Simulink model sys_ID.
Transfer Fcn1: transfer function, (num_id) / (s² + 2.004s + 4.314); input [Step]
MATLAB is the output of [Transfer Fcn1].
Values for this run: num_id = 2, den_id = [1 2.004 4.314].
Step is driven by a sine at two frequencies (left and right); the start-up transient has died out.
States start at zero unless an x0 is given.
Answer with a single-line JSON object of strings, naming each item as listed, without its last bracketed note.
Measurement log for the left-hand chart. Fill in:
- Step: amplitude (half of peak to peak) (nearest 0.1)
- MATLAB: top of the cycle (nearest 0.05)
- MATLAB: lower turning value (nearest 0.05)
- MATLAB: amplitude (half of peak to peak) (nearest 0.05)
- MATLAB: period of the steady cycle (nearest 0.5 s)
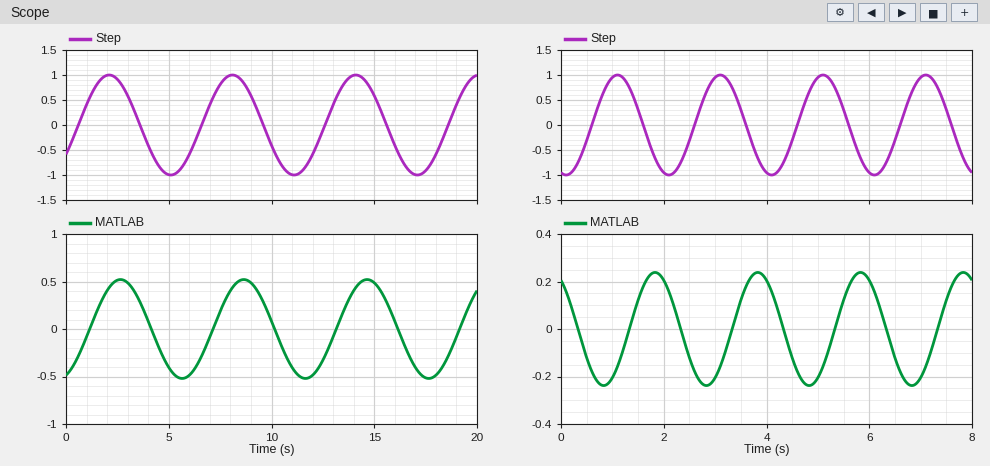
{"Step: amplitude (half of peak to peak)": "1.0", "MATLAB: top of the cycle": "0.50", "MATLAB: lower turning value": "-0.50", "MATLAB: amplitude (half of peak to peak)": "0.50", "MATLAB: period of the steady cycle": "6.0 s"}
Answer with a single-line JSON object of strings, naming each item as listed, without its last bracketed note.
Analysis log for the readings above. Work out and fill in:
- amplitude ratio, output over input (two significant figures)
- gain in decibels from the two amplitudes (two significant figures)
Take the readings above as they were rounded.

{"amplitude ratio, output over input": "0.50", "gain in decibels from the two amplitudes": "-6.0 dB"}
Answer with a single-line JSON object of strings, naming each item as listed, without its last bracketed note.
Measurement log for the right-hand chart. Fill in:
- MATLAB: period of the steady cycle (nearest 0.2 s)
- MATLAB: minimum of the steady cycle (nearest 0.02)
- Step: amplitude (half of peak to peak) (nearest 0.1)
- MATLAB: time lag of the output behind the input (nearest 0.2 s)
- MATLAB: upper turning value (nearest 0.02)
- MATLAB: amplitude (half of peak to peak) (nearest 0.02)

{"MATLAB: period of the steady cycle": "2.0 s", "MATLAB: minimum of the steady cycle": "-0.24", "Step: amplitude (half of peak to peak)": "1.0", "MATLAB: time lag of the output behind the input": "0.8 s", "MATLAB: upper turning value": "0.24", "MATLAB: amplitude (half of peak to peak)": "0.24"}
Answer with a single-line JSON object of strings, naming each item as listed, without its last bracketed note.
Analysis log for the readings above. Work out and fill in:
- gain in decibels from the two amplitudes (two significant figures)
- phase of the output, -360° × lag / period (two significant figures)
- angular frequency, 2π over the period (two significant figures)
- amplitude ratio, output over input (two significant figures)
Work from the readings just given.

{"gain in decibels from the two amplitudes": "-12 dB", "phase of the output, -360° × lag / period": "-140°", "angular frequency, 2π over the period": "3.1 rad/s", "amplitude ratio, output over input": "0.24"}
